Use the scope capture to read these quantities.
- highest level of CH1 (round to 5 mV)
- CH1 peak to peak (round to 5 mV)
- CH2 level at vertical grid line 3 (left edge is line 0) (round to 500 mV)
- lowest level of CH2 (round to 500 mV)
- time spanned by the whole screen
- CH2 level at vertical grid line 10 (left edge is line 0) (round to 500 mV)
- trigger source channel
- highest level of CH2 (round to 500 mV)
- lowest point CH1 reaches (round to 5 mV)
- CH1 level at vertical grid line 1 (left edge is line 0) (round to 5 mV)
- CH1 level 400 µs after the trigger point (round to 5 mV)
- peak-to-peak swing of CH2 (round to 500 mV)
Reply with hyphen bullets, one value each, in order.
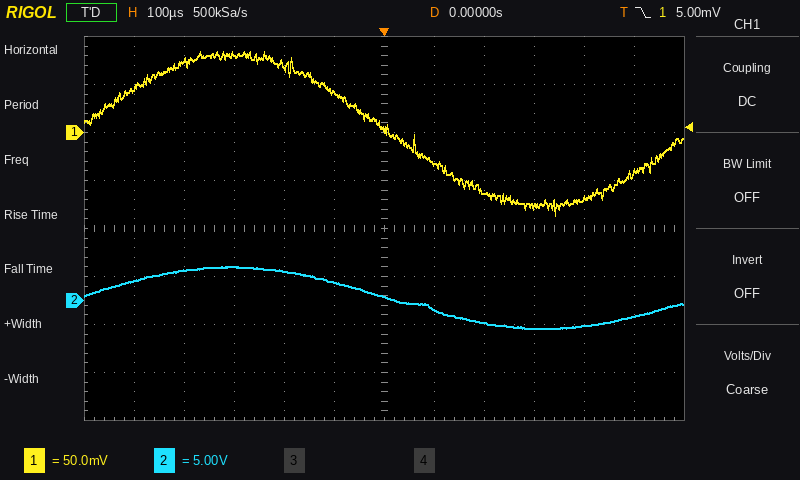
- 85 mV
- 170 mV
- 3.5 V
- -3.0 V
- 1.2 ms
- -2.5 V
- CH1
- 3.5 V
- -85 mV
- 45 mV
- -70 mV
- 6.5 V
